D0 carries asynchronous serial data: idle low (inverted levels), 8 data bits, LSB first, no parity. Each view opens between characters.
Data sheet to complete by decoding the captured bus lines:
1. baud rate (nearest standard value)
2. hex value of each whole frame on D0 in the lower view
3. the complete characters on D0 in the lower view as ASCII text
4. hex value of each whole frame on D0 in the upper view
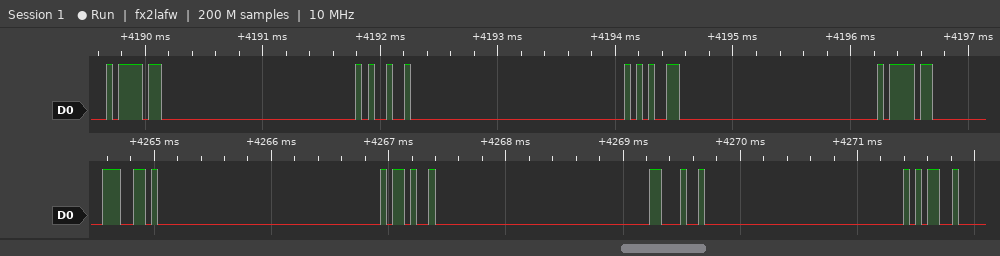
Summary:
19200 baud
4C, 69, 6E, 65
"Line"
21, 6D, 35, 21
